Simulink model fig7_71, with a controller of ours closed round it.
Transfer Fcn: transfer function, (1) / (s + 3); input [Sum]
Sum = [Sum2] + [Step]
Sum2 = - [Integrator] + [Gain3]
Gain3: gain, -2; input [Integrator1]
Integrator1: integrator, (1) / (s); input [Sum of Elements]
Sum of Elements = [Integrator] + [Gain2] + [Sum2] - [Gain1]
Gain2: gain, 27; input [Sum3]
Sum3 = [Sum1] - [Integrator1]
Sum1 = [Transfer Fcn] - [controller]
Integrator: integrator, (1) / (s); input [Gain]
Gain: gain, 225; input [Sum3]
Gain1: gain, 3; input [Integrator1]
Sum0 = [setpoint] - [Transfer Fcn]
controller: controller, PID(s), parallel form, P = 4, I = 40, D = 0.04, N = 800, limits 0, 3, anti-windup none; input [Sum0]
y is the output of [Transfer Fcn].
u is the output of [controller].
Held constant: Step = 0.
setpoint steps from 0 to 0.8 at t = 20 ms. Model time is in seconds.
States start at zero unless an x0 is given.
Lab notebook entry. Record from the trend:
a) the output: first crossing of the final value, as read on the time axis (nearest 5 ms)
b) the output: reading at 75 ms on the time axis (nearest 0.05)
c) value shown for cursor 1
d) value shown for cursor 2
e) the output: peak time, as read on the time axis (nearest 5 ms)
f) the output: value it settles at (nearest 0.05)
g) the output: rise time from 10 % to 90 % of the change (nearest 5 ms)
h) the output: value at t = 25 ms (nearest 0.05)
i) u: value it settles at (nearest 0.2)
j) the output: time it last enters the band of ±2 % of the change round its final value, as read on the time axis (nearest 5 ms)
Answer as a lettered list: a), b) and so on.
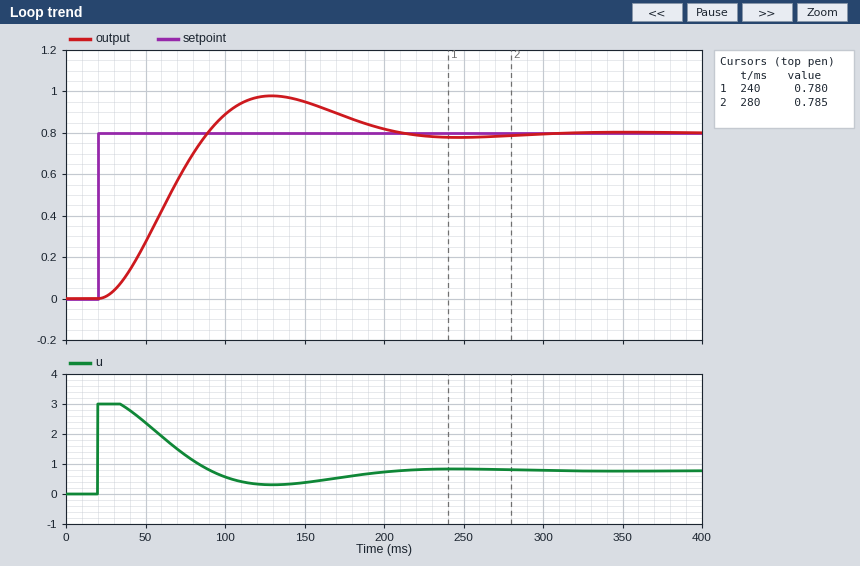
a) 90 ms
b) 0.65
c) 0.780
d) 0.785
e) 130 ms
f) 0.80
g) 45 ms
h) 0.00
i) 0.8
j) 275 ms
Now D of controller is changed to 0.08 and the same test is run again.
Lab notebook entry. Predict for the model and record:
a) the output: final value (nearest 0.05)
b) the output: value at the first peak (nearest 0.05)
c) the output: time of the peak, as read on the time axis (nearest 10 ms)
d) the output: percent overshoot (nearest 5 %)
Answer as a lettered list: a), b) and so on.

a) 0.80
b) 0.95
c) 150 ms
d) 15 %
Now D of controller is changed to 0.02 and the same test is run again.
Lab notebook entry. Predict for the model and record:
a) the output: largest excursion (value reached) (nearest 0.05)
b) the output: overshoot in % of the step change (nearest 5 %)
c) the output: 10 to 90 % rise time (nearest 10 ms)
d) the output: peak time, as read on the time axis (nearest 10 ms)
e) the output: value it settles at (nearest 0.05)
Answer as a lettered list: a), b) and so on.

a) 1.00
b) 25 %
c) 40 ms
d) 120 ms
e) 0.80
